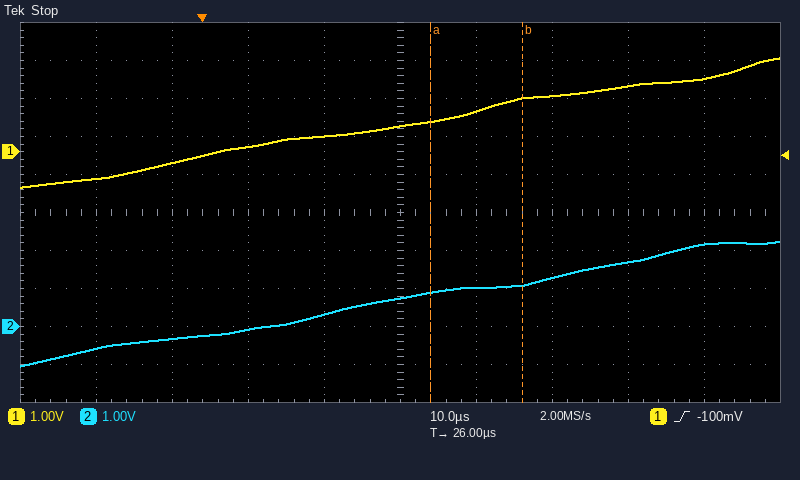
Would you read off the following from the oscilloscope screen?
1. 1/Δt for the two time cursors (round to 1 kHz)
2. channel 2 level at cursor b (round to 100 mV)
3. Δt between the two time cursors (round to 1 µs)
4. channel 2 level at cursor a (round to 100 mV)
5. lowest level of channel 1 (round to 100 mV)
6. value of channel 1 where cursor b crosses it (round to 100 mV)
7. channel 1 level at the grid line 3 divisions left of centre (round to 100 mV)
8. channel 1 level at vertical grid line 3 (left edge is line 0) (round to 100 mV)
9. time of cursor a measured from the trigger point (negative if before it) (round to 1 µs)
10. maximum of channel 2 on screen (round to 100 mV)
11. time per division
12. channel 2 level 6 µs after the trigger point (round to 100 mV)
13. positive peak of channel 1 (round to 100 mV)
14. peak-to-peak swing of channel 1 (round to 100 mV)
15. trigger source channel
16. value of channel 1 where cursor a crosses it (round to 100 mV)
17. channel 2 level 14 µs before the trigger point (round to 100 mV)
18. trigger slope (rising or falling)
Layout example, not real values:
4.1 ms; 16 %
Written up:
83 kHz; 1.1 V; 12 µs; 900 mV; -900 mV; 1.4 V; -300 mV; 100 mV; +30 µs; 2.2 V; 10 µs; -100 mV; 2.5 V; 3.4 V; channel 1; 800 mV; -600 mV; rising
